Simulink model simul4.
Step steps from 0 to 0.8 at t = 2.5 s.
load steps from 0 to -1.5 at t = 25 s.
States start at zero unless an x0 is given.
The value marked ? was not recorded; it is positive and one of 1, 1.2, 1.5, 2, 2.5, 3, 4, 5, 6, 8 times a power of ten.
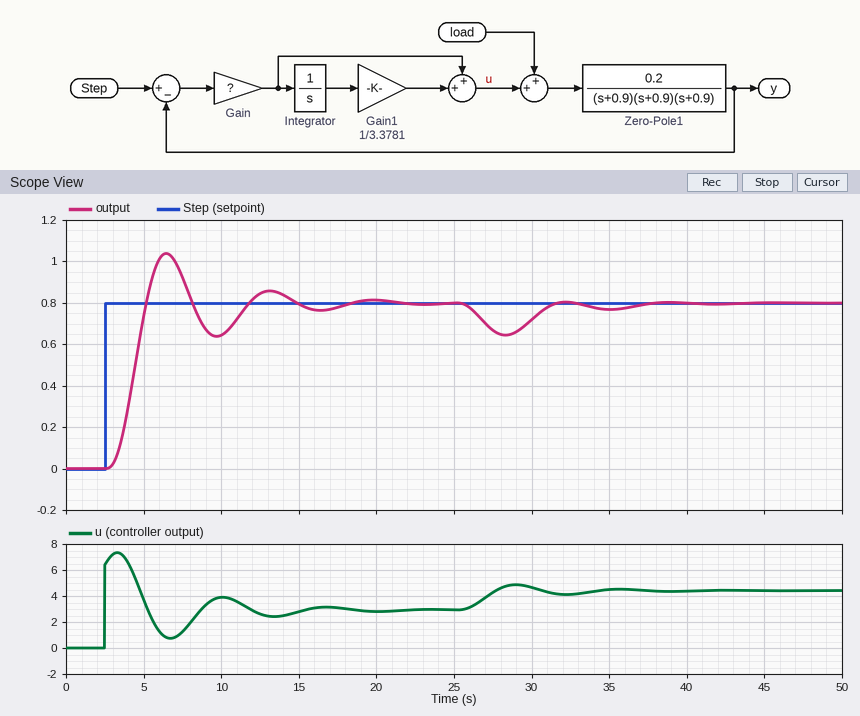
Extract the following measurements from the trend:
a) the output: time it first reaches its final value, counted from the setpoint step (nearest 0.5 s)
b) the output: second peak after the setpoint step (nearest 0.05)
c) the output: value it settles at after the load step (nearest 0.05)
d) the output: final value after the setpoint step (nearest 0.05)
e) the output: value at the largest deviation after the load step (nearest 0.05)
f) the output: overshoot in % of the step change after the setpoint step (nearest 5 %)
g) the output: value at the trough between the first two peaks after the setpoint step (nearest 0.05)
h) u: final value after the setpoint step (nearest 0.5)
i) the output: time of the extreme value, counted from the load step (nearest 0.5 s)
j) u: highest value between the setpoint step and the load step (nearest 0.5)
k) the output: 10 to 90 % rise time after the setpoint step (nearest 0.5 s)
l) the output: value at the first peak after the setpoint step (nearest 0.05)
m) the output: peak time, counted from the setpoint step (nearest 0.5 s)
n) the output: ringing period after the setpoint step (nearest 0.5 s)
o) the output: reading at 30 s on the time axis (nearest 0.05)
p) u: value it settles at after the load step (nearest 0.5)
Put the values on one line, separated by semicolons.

2.5 s; 0.85; 0.80; 0.80; 0.65; 30 %; 0.65; 3.0; 3.5 s; 7.5; 1.5 s; 1.05; 4.0 s; 6.5 s; 0.70; 4.5
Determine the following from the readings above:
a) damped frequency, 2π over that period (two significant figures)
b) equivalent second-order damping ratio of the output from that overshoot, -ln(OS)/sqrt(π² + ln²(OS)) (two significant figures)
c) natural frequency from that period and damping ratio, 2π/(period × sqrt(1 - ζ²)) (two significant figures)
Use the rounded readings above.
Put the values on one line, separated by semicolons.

0.97 rad/s; 0.36; 1.0 rad/s
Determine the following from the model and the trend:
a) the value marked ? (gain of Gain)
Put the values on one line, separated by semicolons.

8
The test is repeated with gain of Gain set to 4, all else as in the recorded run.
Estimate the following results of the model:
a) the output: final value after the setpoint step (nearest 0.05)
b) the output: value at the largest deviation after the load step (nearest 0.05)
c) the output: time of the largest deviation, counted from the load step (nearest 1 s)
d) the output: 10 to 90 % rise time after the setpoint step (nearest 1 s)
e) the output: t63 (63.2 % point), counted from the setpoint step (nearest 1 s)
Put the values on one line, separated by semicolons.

0.80; 0.60; 4 s; 3 s; 3 s
